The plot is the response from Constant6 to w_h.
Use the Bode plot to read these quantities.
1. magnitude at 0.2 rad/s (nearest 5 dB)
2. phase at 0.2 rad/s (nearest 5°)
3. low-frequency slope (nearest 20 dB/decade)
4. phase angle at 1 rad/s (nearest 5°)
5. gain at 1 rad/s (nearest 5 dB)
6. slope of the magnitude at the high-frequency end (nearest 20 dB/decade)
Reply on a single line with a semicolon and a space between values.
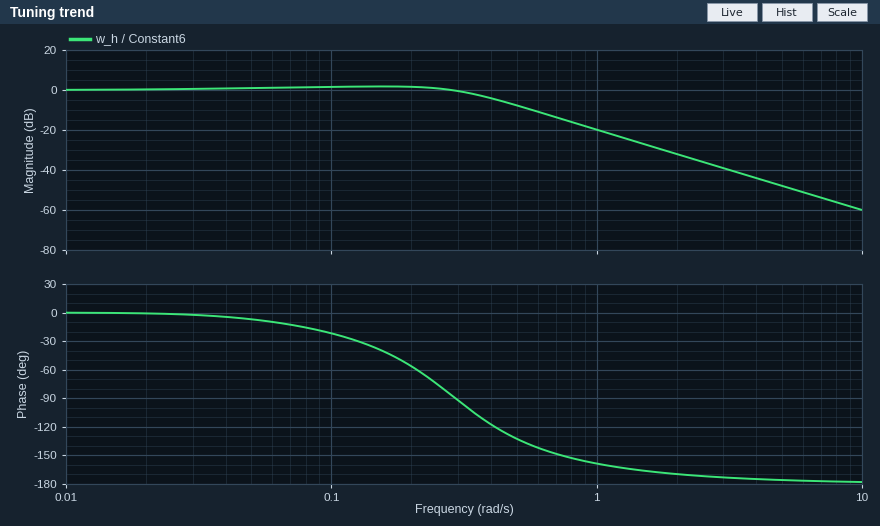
0 dB; -55°; 0 dB/decade; -160°; -20 dB; -40 dB/decade
